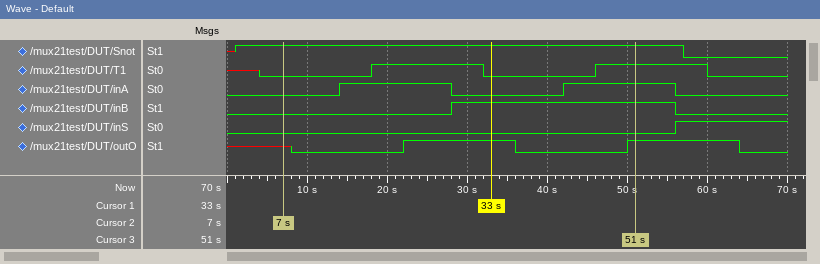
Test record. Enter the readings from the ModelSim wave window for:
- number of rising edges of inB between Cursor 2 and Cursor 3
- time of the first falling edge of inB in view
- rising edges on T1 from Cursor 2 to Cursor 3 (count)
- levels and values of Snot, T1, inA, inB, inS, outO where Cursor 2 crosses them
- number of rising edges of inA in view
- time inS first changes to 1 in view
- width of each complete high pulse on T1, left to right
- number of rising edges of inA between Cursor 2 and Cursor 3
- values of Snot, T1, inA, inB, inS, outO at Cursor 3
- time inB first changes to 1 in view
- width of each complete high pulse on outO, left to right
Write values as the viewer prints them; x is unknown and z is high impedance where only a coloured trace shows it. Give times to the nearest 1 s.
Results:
1
56 s
2
Snot=1, T1=0, inA=0, inB=0, inS=0, outO=x
2
56 s
14 s, 14 s
2
Snot=1, T1=1, inA=1, inB=1, inS=0, outO=1
28 s
14 s, 14 s
